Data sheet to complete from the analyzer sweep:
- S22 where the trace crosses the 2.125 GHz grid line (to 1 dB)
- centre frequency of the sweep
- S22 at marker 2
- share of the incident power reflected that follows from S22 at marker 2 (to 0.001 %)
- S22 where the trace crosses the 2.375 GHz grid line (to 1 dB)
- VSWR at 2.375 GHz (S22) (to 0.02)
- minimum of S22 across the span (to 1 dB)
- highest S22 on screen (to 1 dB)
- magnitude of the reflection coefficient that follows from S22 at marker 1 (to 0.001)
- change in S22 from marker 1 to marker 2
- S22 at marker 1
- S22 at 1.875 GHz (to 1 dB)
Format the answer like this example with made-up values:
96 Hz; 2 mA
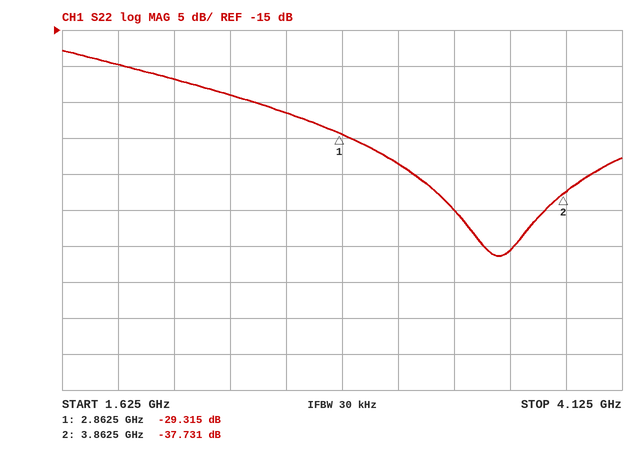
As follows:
-22 dB; 2.875 GHz; -37.731 dB; 0.017 %; -24 dB; 1.14; -46 dB; -18 dB; 0.034; -8.416 dB; -29.315 dB; -20 dB
